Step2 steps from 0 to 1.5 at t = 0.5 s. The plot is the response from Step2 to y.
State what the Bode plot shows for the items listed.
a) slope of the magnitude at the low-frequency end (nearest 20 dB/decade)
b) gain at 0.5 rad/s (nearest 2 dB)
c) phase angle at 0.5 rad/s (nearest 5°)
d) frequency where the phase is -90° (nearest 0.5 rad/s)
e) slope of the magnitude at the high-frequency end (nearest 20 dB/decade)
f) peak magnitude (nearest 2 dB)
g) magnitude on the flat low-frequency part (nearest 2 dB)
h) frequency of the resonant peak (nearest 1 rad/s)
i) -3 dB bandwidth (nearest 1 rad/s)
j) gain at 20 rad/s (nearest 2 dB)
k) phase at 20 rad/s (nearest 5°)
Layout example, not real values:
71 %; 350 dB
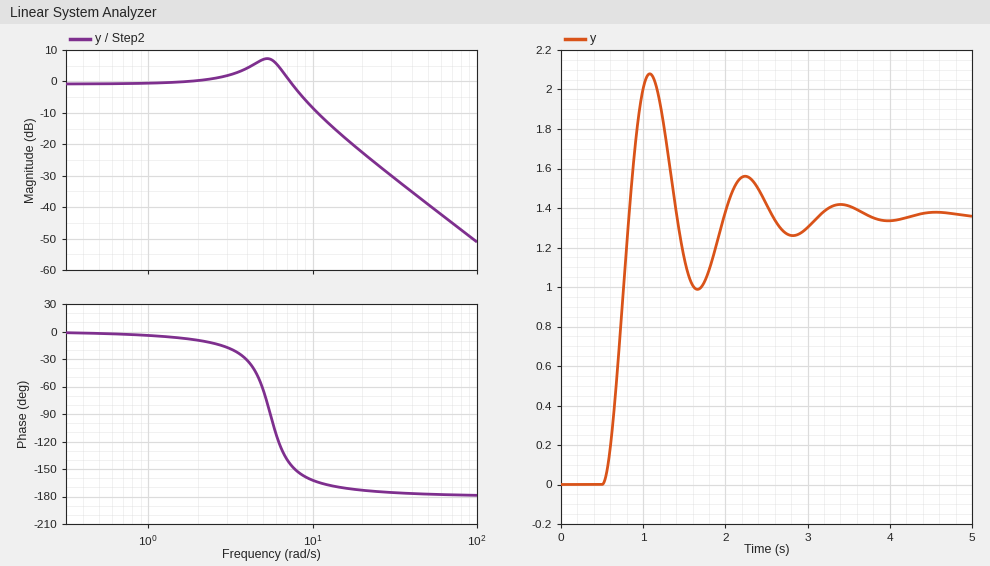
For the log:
0 dB/decade; 0 dB; 0°; 5.5 rad/s; -40 dB/decade; 8 dB; 0 dB; 5 rad/s; 8 rad/s; -22 dB; -175°
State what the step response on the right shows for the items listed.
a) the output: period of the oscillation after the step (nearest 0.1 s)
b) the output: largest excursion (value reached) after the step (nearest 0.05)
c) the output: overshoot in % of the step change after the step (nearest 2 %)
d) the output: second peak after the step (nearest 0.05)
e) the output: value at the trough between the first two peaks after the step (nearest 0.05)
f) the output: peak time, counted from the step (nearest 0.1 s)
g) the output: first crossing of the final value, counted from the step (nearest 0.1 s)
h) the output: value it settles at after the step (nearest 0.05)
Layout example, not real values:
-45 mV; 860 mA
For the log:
1.2 s; 2.10; 52 %; 1.55; 1.00; 0.6 s; 0.3 s; 1.35
